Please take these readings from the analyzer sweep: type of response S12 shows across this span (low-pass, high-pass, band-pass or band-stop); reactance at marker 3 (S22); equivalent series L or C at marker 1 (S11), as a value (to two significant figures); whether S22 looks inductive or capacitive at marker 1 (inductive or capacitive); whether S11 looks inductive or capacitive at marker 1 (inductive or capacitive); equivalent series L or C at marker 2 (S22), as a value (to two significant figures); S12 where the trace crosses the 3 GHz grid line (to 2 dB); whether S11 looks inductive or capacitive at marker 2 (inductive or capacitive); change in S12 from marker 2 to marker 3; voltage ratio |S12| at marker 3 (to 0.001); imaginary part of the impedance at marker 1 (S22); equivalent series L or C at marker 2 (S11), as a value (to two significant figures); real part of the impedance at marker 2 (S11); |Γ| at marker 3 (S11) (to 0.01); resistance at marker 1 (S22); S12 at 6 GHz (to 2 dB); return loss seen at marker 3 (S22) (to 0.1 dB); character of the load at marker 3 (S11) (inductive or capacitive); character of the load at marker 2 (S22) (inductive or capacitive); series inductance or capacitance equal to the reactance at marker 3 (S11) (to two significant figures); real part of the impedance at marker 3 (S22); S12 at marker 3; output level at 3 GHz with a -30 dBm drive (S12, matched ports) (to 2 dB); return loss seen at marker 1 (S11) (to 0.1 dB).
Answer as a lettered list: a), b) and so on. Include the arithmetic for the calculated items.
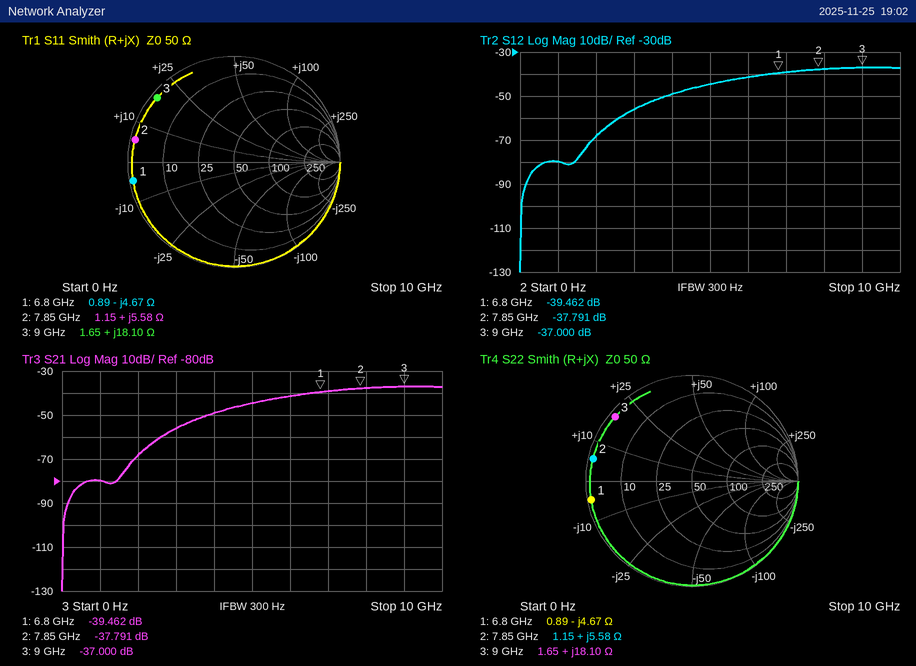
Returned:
a) high-pass
b) +18.10 Ω
c) C = 1/(2π × 6.8 GHz × 4.67 Ω) ≈ 5.0 pF
d) capacitive
e) capacitive
f) L = 5.58 Ω/(2π × 7.85 GHz) ≈ 113 pH, so 110 pH to two significant figures
g) -56 dB
h) inductive
i) -37 − (-37.791) = 0.791 dB
j) 10^(-37/20) ≈ 0.014
k) -4.67 Ω
l) L = 5.58 Ω/(2π × 7.85 GHz) ≈ 113 pH, so 110 pH to two significant figures
m) 1.15 Ω
n) 0.94
o) 0.89 Ω
p) -42 dB
q) 0.5 dB
r) inductive
s) inductive
t) L = 18.1 Ω/(2π × 9 GHz) ≈ 320 pH
u) 1.65 Ω
v) -37.000 dB
w) -30 dBm + (-56 dB) = -86 dBm
x) 0.3 dB
